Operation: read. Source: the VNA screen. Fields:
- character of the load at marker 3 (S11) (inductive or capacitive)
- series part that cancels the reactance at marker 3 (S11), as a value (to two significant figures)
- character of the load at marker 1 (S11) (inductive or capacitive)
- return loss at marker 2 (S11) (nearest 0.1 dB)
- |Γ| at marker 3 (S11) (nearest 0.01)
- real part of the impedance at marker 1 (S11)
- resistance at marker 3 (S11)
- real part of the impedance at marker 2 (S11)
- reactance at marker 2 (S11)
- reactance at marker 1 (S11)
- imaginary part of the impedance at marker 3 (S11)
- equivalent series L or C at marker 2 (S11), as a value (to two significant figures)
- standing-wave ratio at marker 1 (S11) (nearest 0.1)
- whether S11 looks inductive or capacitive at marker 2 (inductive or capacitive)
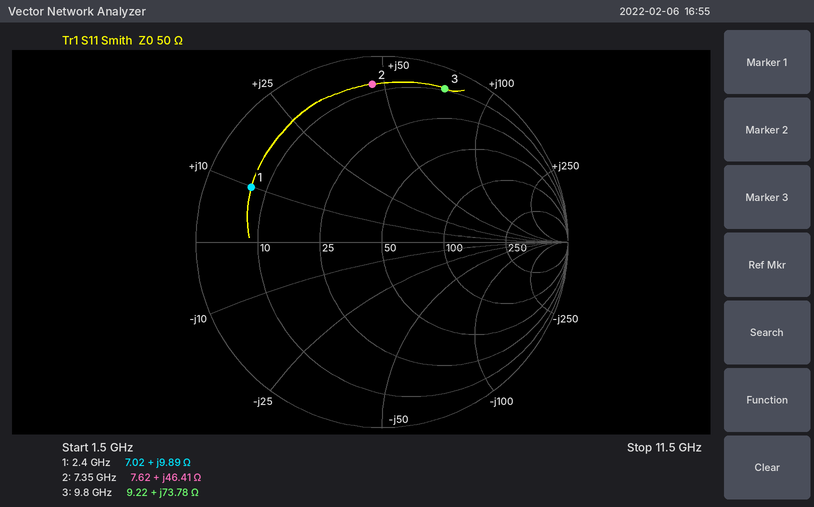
inductive
220 fF
inductive
1.4 dB
0.89
7.02 Ω
9.22 Ω
7.62 Ω
+46.41 Ω
+9.89 Ω
+73.78 Ω
1.0 nH
7.4
inductive
